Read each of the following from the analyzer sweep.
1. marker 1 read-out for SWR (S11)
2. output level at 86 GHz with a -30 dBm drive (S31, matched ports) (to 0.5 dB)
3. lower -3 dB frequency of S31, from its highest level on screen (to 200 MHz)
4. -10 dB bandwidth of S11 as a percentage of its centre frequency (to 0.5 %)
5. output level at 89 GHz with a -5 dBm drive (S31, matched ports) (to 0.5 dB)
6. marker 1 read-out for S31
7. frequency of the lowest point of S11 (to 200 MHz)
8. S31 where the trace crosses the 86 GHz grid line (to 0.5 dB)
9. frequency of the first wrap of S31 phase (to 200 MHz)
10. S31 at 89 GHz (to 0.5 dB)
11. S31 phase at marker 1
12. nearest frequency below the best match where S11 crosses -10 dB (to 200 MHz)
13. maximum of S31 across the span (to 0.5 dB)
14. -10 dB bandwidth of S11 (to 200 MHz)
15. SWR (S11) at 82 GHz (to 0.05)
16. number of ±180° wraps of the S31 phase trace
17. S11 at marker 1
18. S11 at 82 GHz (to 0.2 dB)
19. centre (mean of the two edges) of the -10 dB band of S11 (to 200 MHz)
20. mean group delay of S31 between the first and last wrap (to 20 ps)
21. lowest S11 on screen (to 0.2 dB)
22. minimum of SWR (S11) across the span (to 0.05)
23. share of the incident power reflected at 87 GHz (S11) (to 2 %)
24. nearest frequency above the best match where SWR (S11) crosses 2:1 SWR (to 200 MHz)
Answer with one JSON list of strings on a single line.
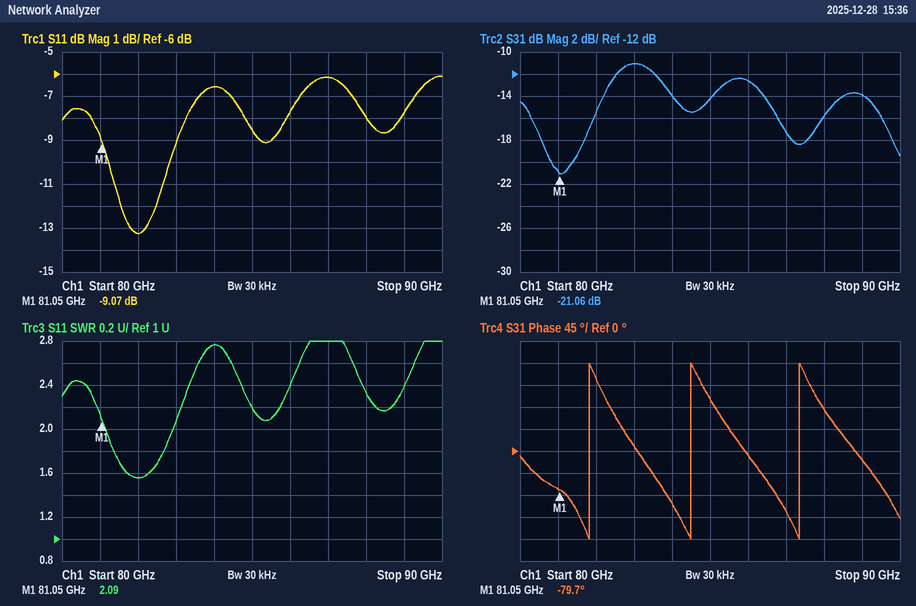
["2.09", "-42.5 dBm", "82.2 GHz", "2.0 %", "-19.0 dBm", "-21.06 dB", "82.0 GHz", "-12.5 dB", "81.8 GHz", "-14.0 dB", "-79.7°", "81.2 GHz", "-11.0 dB", "1.6 GHz", "1.55", "3", "-9.07 dB", "-13.2 dB", "82.0 GHz", "360 ps", "-13.2 dB", "1.55", "24 %", "83.0 GHz"]
